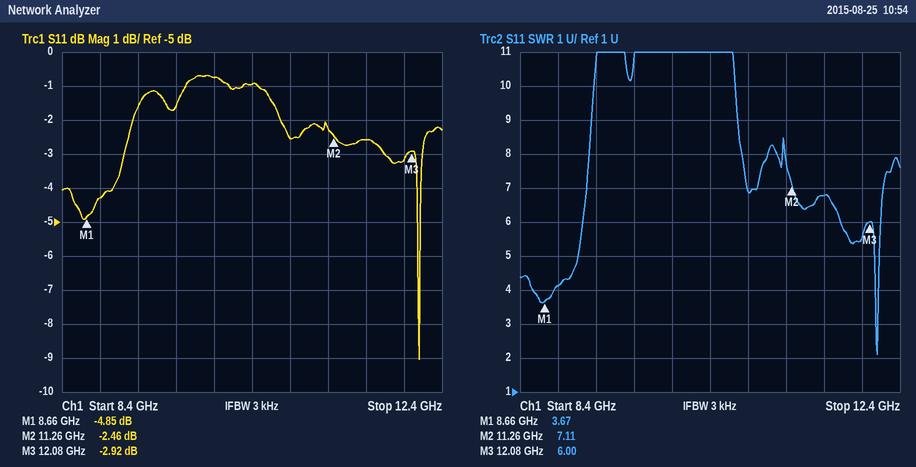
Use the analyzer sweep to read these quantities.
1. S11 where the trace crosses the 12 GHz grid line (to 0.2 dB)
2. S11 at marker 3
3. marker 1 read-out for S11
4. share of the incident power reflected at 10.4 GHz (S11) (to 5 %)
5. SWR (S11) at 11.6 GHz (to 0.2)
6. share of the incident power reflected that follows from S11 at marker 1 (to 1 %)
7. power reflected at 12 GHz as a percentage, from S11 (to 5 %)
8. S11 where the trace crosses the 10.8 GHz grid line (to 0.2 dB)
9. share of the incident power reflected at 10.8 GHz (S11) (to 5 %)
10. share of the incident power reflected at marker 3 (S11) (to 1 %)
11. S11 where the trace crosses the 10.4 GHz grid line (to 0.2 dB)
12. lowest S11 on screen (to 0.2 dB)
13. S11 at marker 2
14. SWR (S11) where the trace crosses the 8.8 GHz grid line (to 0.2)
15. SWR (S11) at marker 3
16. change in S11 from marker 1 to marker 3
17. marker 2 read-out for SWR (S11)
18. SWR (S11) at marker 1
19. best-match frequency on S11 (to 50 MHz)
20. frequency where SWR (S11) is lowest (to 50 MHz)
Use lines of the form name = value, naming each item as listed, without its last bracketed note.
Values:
S11 where the trace crosses the 12 GHz grid line = -3.2 dB
S11 at marker 3 = -2.92 dB
marker 1 read-out for S11 = -4.85 dB
share of the incident power reflected at 10.4 GHz (S11) = 80 %
SWR (S11) at 11.6 GHz = 6.8
share of the incident power reflected that follows from S11 at marker 1 = 33 %
power reflected at 12 GHz as a percentage, from S11 = 50 %
S11 where the trace crosses the 10.8 GHz grid line = -2.6 dB
share of the incident power reflected at 10.8 GHz (S11) = 55 %
share of the incident power reflected at marker 3 (S11) = 51 %
S11 where the trace crosses the 10.4 GHz grid line = -1.0 dB
lowest S11 on screen = -9.0 dB
S11 at marker 2 = -2.46 dB
SWR (S11) where the trace crosses the 8.8 GHz grid line = 4.2
SWR (S11) at marker 3 = 6.00
change in S11 from marker 1 to marker 3 = 1.93 dB
marker 2 read-out for SWR = 7.11
SWR (S11) at marker 1 = 3.67
best-match frequency on S11 = 12.15 GHz
frequency where SWR (S11) is lowest = 12.15 GHz
